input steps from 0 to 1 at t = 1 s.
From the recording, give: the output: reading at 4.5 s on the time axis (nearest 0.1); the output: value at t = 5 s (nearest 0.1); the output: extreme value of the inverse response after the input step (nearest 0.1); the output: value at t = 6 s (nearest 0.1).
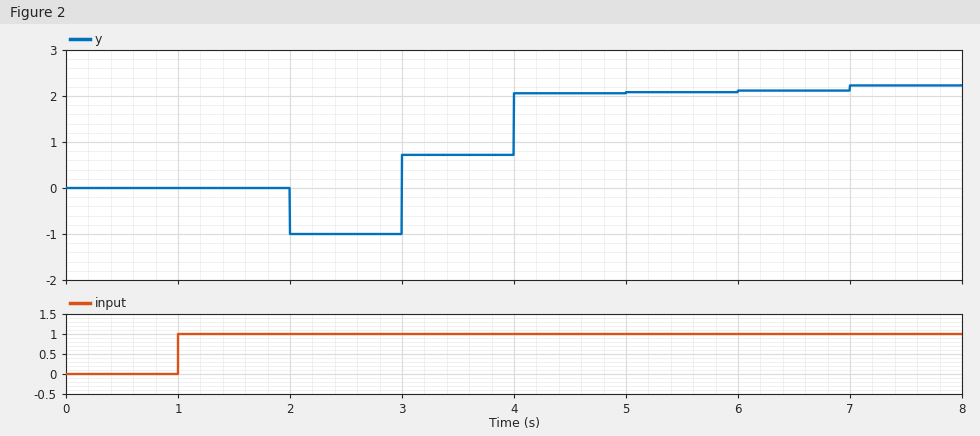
2.1
2.1
-1.0
2.1
